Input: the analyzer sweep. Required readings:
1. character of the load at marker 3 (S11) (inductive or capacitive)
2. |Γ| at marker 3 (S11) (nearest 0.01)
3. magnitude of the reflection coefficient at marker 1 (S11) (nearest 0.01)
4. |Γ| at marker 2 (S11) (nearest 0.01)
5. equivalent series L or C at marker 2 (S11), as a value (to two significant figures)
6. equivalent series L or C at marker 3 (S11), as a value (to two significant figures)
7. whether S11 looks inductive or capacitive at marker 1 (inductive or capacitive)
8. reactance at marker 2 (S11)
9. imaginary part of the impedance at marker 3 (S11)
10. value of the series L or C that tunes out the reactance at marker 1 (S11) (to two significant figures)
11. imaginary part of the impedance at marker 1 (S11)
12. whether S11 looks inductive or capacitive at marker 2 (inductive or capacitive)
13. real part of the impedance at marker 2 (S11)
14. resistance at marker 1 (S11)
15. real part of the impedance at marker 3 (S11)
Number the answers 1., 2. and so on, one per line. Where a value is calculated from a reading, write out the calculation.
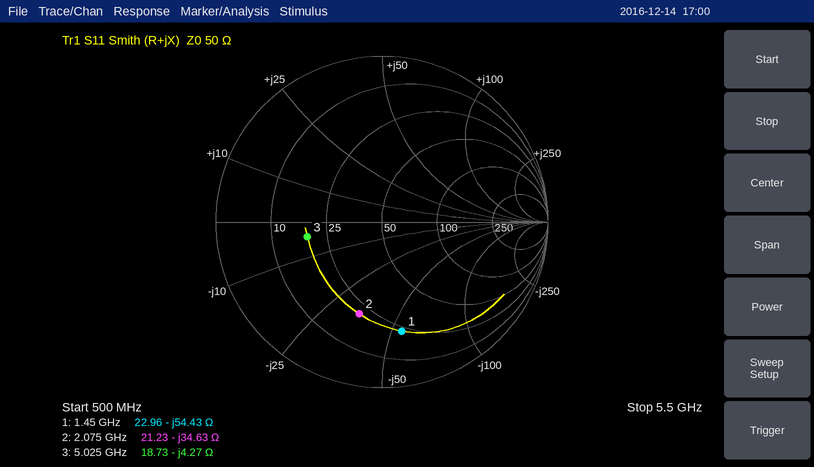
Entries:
1. capacitive
2. 0.46
3. 0.67
4. 0.57
5. C = 1/(2π × 2.075 GHz × 34.63 Ω) ≈ 2.2 pF
6. C = 1/(2π × 5.025 GHz × 4.27 Ω) ≈ 7.4 pF
7. capacitive
8. -34.63 Ω
9. -4.27 Ω
10. L = 54.43 Ω/(2π × 1.45 GHz) ≈ 6.0 nH
11. -54.43 Ω
12. capacitive
13. 21.23 Ω
14. 22.96 Ω
15. 18.73 Ω
